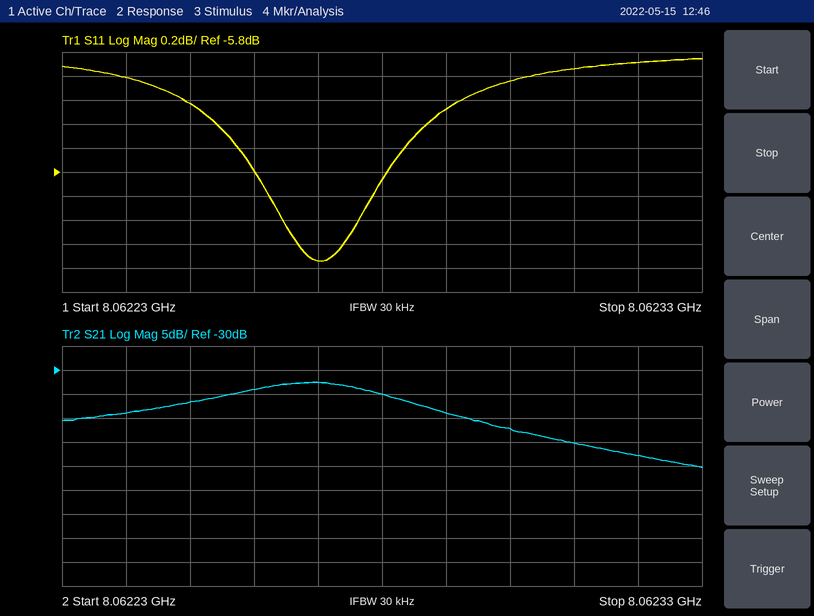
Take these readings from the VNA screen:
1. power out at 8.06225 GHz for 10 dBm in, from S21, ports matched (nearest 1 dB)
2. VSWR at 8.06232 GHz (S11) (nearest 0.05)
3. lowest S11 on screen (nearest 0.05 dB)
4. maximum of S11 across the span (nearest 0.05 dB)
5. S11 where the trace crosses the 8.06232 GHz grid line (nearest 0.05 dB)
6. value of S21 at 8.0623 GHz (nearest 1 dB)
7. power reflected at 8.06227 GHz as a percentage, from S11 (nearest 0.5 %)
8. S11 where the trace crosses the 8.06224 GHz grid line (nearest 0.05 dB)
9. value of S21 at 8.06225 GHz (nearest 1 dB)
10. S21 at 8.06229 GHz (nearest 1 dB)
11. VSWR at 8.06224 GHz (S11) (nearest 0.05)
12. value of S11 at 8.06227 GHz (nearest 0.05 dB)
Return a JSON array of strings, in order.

["-27 dBm", "3.65", "-6.55 dB", "-4.85 dB", "-4.90 dB", "-42 dB", "22.0 %", "-5.00 dB", "-37 dB", "-39 dB", "3.55", "-6.55 dB"]
